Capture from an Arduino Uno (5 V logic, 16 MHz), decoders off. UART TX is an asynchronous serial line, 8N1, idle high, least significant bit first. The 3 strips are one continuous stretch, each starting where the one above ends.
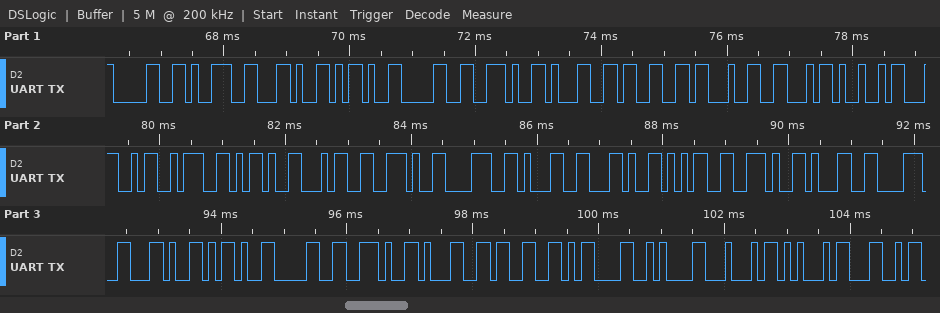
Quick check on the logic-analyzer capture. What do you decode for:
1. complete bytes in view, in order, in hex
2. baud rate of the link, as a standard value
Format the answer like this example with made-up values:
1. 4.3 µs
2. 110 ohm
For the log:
1. 0x30 0x39 0x2C 0x2D 0x30 0x2E 0x31 0x33 0x23 0x46 0x49 0x4C 0x3A 0x2D 0x34 0x2E 0x38 0x31 0x2C 0x35 0x2E 0x31 0x38 0x2C 0x2D 0x30 0x2E 0x31 0x33 0x0D 0x0A 0x44 0x45 0x4C
2. 9600 baud
